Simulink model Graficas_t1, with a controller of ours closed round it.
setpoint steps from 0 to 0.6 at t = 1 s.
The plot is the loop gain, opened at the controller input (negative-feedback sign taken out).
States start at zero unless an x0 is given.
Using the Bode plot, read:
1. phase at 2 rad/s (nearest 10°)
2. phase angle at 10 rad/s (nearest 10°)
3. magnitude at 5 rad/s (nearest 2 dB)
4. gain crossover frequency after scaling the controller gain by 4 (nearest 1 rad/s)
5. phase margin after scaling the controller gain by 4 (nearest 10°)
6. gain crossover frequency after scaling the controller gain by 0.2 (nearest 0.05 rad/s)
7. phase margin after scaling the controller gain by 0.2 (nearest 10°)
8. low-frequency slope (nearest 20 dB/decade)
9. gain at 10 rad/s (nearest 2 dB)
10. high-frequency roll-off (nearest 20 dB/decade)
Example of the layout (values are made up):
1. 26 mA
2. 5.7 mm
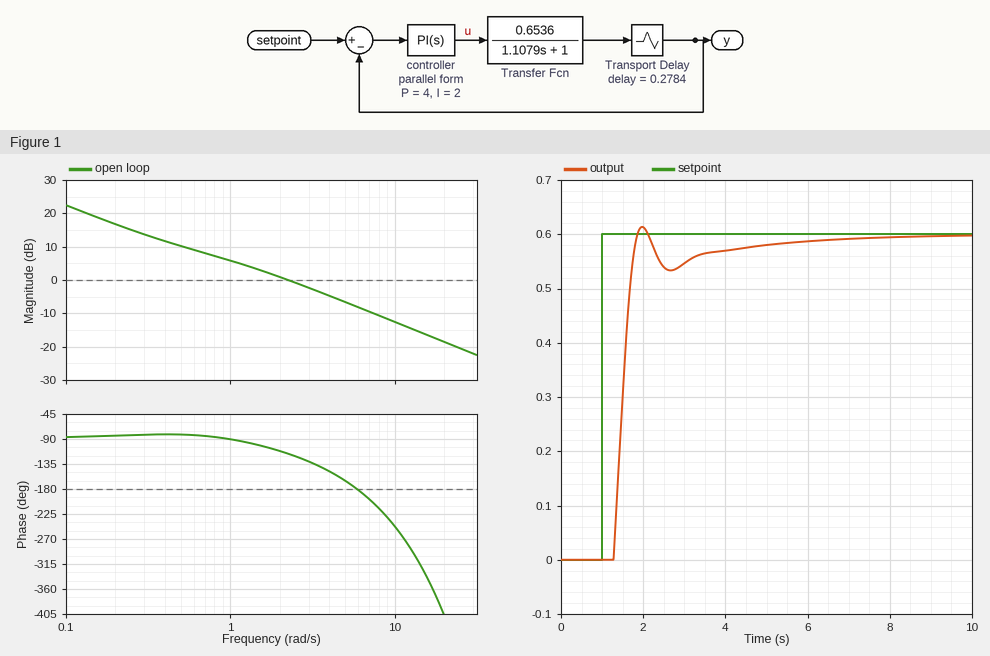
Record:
1. -110°
2. -250°
3. -6 dB
4. 9 rad/s
5. -60°
6. 0.30 rad/s
7. 100°
8. -20 dB/decade
9. -12 dB
10. -20 dB/decade
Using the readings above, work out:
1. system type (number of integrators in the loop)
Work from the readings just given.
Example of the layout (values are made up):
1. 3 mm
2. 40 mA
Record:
1. 1
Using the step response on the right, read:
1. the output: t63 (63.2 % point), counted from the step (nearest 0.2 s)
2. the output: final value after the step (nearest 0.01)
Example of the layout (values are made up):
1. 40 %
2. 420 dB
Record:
1. 0.6 s
2. 0.60
